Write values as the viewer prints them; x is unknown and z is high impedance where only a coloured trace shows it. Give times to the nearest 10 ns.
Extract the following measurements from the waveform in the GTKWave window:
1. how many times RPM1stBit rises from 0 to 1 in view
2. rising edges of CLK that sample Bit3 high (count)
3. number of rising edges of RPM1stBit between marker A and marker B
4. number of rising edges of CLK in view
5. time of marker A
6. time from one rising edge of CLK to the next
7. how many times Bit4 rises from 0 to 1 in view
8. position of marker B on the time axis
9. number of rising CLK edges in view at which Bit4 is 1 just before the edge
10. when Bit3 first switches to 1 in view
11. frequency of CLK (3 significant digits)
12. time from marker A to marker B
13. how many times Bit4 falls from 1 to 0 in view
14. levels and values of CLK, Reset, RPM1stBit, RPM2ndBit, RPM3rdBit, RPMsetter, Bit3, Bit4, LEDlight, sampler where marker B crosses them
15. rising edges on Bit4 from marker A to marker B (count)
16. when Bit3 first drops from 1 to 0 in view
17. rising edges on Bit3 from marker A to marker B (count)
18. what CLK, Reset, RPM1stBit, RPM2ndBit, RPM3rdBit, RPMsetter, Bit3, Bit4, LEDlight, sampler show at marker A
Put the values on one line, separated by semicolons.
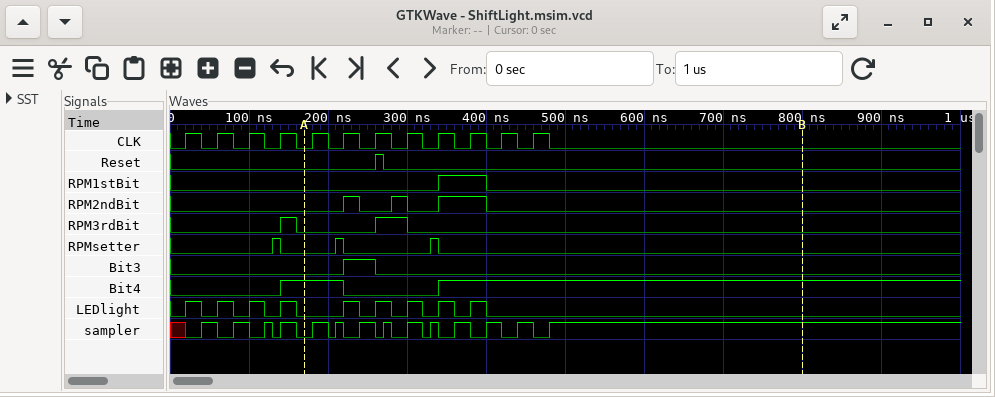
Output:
1; 1; 1; 12; 170 ns; 40 ns; 2; 800 ns; 5; 220 ns; 25.0 MHz; 630 ns; 1; CLK=0, Reset=0, RPM1stBit=0, RPM2ndBit=0, RPM3rdBit=0, RPMsetter=0, Bit3=0, Bit4=1, LEDlight=0, sampler=1; 1; 260 ns; 1; CLK=0, Reset=0, RPM1stBit=0, RPM2ndBit=0, RPM3rdBit=0, RPMsetter=0, Bit3=0, Bit4=1, LEDlight=0, sampler=0
